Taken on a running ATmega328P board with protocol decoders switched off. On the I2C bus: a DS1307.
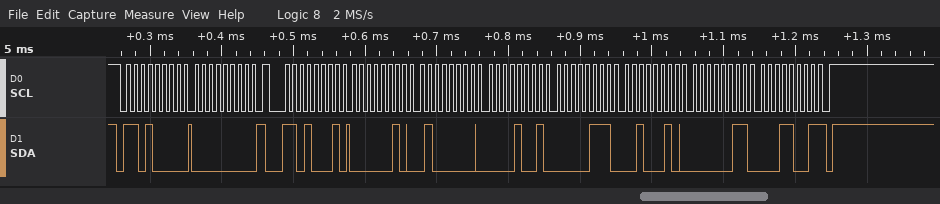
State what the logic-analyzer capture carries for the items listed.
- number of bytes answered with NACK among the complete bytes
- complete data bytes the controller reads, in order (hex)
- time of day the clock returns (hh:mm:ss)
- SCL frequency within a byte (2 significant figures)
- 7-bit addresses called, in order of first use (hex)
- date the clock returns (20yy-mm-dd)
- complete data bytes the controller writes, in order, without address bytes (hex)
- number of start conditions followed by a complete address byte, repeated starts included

1
02 40 09 07 22 03 19
09:40:02
100 kHz
0x68
2019-03-22
00
2
